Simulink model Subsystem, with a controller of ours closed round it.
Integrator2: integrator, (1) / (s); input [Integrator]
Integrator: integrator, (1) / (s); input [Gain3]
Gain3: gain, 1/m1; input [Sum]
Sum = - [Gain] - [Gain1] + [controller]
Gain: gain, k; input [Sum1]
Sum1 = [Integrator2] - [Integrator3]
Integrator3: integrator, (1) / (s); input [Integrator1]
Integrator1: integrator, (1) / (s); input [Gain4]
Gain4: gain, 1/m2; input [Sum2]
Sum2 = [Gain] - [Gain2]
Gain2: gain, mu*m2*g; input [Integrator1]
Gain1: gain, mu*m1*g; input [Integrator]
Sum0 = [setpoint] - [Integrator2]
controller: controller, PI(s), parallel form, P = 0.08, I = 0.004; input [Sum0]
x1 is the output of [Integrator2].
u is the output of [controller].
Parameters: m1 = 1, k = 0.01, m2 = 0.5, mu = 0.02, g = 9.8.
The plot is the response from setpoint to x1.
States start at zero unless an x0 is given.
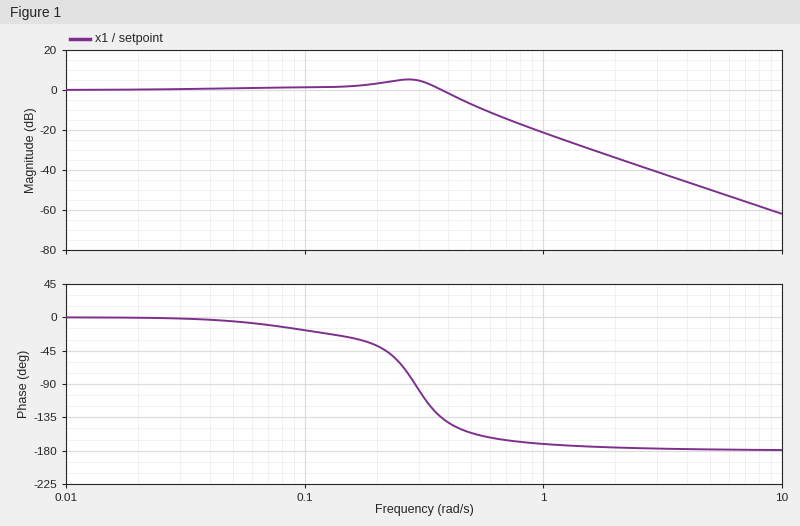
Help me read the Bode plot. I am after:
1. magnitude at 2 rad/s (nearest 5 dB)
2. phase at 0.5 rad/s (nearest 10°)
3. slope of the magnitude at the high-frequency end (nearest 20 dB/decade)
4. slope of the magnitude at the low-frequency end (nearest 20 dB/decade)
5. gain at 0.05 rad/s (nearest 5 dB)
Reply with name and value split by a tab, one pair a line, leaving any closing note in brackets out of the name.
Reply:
magnitude at 2 rad/s	-35 dB
phase at 0.5 rad/s	-160°
slope of the magnitude at the high-frequency end	-40 dB/decade
slope of the magnitude at the low-frequency end	0 dB/decade
gain at 0.05 rad/s	0 dB
